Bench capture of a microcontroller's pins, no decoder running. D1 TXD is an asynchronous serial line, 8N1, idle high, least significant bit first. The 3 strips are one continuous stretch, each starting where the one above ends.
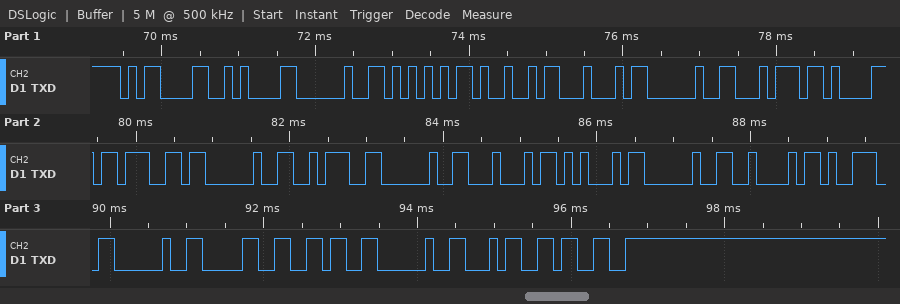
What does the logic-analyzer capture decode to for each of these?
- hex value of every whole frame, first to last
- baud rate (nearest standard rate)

0D 0A 20 55 49 44 20 74 61 67 20 3A 20 44 45 20 42 39 20 30 36 20 34 33
9600 baud
